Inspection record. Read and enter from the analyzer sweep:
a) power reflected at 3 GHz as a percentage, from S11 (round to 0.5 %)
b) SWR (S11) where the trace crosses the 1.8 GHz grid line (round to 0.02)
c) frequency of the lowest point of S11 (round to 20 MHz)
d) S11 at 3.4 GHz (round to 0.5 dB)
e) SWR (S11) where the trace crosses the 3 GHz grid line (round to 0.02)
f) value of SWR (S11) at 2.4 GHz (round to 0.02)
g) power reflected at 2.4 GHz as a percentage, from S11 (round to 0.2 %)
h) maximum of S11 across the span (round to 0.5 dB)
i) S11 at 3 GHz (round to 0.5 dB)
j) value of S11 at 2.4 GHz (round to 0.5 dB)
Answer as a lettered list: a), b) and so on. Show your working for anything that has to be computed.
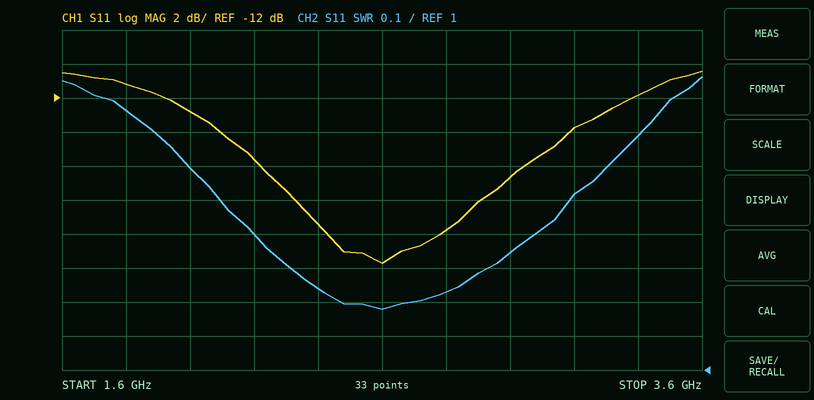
a) 10^(-16.5/10) ≈ 2.24 %, so 2.0 % to the nearest 0.5 %
b) 1.76
c) 2.60 GHz
d) -12.0 dB
e) 1.34
f) 1.24
g) 10^(-19.5/10) ≈ 1.12 %, so 1.2 % to the nearest 0.2 %
h) -10.5 dB
i) -16.5 dB
j) -19.5 dB
